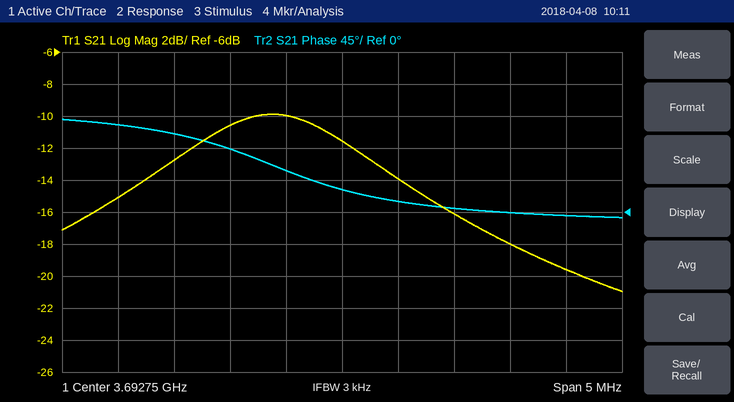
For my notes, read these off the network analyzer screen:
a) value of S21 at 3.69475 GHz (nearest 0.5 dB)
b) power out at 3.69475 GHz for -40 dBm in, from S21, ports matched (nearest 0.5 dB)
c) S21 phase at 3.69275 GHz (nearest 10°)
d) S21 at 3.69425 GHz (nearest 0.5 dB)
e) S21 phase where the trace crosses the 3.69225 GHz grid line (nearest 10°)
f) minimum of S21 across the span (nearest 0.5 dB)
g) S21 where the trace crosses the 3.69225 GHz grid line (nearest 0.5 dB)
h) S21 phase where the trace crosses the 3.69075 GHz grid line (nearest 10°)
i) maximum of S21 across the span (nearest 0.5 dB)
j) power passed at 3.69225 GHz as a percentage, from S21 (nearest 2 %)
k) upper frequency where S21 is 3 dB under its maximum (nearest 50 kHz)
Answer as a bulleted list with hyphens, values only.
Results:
- -19.5 dB
- -59.5 dBm
- 30°
- -18.0 dB
- 60°
- -21.0 dB
- -10.0 dB
- 120°
- -10.0 dB
- 10 %
- 3.69305 GHz
